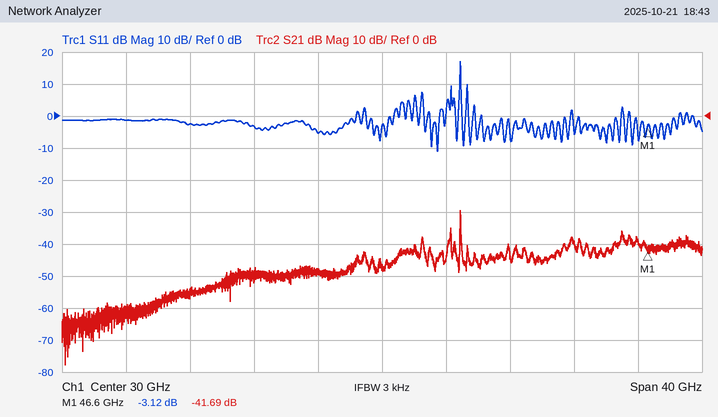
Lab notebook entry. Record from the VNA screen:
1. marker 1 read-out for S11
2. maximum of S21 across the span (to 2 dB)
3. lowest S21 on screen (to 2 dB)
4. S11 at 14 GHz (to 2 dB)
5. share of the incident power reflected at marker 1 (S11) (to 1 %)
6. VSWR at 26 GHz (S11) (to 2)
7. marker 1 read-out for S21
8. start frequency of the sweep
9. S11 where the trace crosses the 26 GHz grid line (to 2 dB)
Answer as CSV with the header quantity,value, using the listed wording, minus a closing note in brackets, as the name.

quantity,value
marker 1 read-out for S11,-3.12 dB
maximum of S21 across the span,-30 dB
lowest S21 on screen,-78 dB
S11 at 14 GHz,-2 dB
share of the incident power reflected at marker 1 (S11),49 %
VSWR at 26 GHz (S11),4
marker 1 read-out for S21,-41.69 dB
start frequency of the sweep,10 GHz
S11 where the trace crosses the 26 GHz grid line,-6 dB
